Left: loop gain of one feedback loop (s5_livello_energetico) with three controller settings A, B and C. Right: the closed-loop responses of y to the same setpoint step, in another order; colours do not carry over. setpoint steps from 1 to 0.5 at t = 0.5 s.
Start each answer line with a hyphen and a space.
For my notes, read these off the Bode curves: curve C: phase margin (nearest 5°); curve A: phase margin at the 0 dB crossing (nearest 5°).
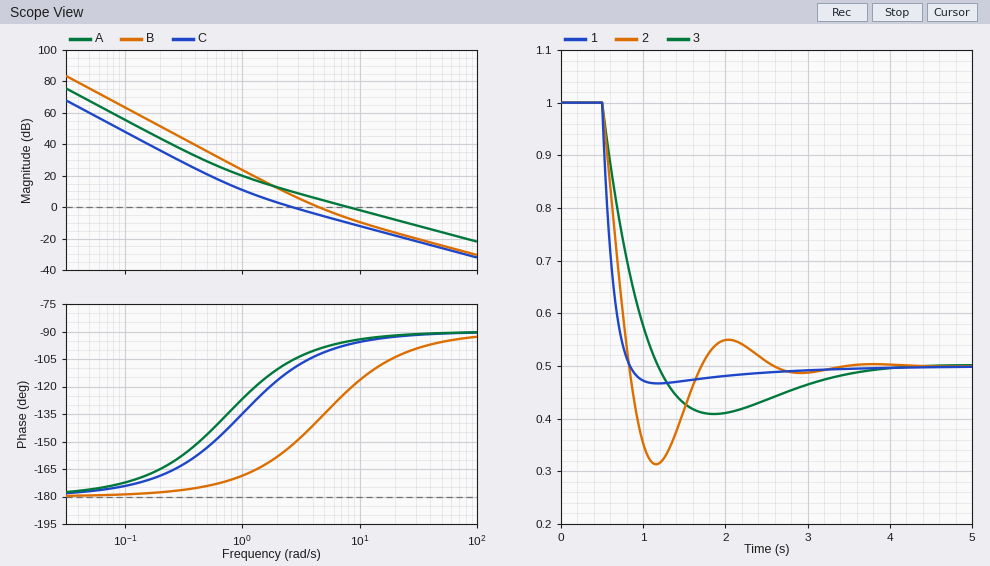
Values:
- 70°
- 85°
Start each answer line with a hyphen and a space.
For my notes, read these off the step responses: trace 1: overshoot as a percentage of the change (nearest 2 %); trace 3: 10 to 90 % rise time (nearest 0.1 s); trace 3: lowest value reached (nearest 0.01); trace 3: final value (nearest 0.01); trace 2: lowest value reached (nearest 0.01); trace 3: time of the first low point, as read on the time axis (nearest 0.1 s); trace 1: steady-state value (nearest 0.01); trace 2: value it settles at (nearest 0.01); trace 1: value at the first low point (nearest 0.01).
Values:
- 6 %
- 0.5 s
- 0.41
- 0.50
- 0.31
- 1.9 s
- 0.50
- 0.50
- 0.47
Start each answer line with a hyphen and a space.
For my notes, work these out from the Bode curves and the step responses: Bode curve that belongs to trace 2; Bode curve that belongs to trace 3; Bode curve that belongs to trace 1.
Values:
- B
- C
- A
